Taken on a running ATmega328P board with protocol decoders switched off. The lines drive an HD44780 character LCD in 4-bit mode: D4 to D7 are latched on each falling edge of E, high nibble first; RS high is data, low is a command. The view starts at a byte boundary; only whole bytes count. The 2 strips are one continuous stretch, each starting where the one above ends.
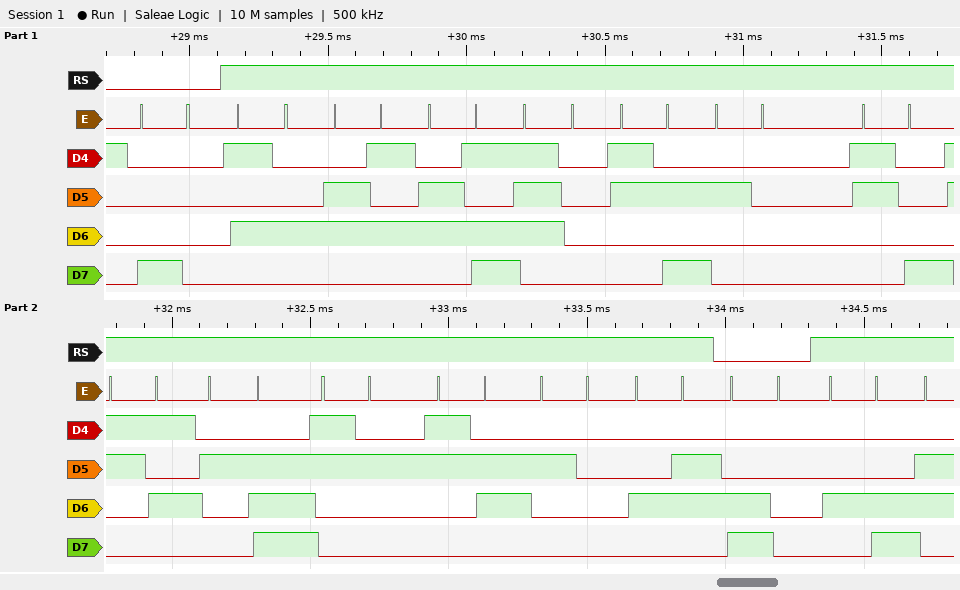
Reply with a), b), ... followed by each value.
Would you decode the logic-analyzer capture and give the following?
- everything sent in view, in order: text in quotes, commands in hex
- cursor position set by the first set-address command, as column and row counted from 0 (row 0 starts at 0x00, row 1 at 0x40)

a) 0x80 "Temp: 85.26 F" 0xC0 "L"
b) column 0, row 0
